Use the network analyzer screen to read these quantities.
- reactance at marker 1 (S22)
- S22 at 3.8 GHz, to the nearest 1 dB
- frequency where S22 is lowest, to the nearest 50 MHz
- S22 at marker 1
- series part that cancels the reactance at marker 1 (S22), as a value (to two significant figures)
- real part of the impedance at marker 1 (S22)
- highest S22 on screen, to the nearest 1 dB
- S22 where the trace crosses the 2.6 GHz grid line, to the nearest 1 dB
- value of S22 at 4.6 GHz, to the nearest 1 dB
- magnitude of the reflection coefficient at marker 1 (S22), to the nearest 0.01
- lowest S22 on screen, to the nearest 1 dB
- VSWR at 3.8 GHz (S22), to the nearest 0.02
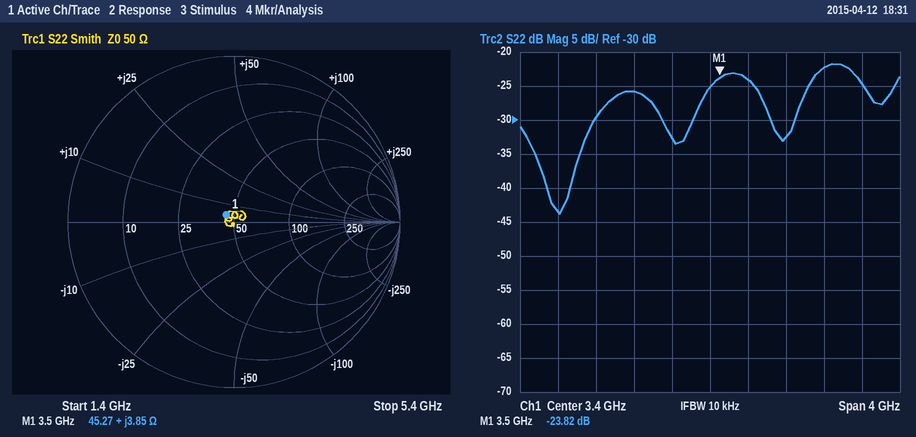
+3.85 Ω
-24 dB
1.80 GHz
-23.82 dB
12 pF
45.27 Ω
-22 dB
-26 dB
-22 dB
0.06
-44 dB
1.14
